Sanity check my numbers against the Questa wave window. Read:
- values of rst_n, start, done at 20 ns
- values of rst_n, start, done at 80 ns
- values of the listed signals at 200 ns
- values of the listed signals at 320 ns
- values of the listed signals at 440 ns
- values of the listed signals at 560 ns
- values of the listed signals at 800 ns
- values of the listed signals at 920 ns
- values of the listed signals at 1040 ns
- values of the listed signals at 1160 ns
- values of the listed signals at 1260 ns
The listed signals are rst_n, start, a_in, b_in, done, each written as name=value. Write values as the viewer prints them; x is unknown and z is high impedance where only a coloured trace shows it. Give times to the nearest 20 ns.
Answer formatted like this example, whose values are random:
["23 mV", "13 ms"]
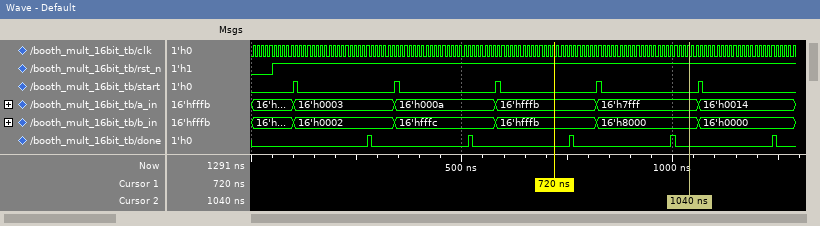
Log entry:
["rst_n=0, start=0, done=0", "rst_n=1, start=0, done=0", "rst_n=1, start=0, a_in=16'h0003, b_in=16'h0002, done=0", "rst_n=1, start=0, a_in=16'h0003, b_in=16'h0002, done=0", "rst_n=1, start=0, a_in=16'h000a, b_in=16'hfffc, done=0", "rst_n=1, start=0, a_in=16'h000a, b_in=16'hfffc, done=0", "rst_n=1, start=0, a_in=16'hfffb, b_in=16'hfffb, done=0", "rst_n=1, start=0, a_in=16'h7fff, b_in=16'h8000, done=0", "rst_n=1, start=0, a_in=16'h7fff, b_in=16'h8000, done=0", "rst_n=1, start=0, a_in=16'h0014, b_in=16'h0000, done=0", "rst_n=1, start=0, a_in=16'h0014, b_in=16'h0000, done=0"]
